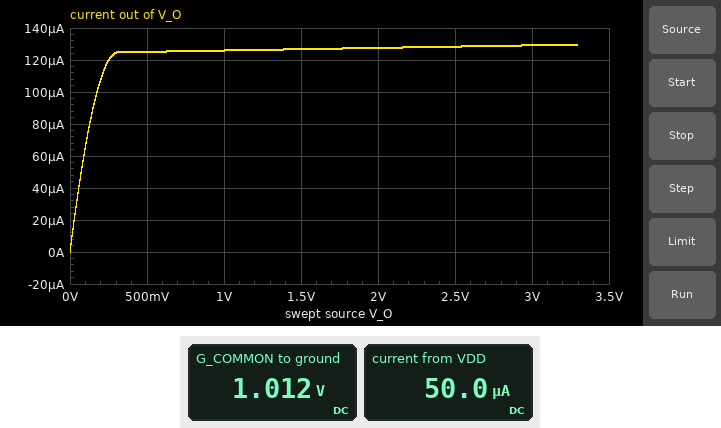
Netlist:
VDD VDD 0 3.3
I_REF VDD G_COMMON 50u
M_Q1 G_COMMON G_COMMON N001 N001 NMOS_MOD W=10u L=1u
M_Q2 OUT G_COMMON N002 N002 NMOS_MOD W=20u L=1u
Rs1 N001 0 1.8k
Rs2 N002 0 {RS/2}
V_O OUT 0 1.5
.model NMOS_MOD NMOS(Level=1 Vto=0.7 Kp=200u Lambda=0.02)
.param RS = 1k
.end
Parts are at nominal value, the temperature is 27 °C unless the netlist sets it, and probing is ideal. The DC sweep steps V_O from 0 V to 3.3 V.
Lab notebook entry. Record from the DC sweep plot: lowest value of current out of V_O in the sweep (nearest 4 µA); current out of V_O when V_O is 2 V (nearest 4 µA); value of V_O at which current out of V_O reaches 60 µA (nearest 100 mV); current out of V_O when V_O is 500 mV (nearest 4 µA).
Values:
0 A
128 µA
100 mV
124 µA
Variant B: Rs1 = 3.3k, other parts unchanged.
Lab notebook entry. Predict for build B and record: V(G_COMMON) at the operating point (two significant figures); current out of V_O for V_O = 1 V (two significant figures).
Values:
1.1 V
180 µA
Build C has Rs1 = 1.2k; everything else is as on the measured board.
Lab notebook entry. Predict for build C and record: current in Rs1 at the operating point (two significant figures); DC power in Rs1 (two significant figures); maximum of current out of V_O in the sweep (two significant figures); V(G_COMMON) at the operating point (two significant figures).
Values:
50 µA
3.0 µW
110 µA
980 mV
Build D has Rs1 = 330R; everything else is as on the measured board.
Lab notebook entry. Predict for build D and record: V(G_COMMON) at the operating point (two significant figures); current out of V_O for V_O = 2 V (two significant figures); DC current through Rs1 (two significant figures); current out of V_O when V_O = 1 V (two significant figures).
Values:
940 mV
81 µA
50 µA
80 µA
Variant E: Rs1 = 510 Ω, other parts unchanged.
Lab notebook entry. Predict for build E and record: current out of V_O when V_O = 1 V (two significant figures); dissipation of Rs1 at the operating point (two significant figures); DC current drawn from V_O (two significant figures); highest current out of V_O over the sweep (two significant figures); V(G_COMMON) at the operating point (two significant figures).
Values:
85 µA
1.3 µW
86 µA
88 µA
950 mV
